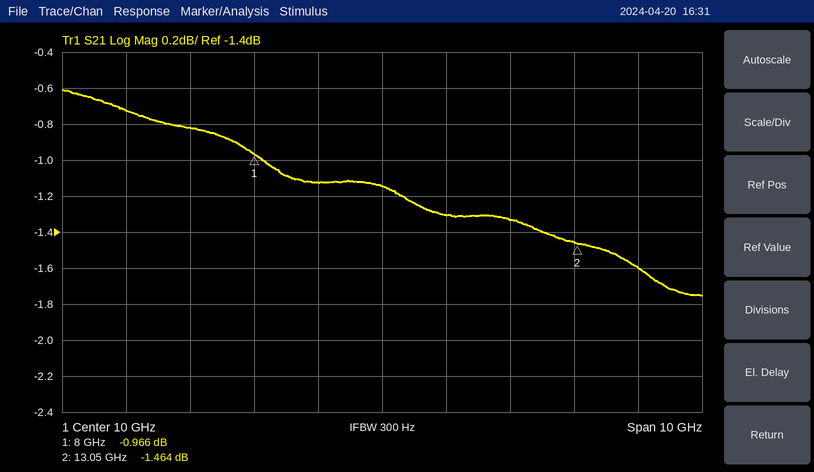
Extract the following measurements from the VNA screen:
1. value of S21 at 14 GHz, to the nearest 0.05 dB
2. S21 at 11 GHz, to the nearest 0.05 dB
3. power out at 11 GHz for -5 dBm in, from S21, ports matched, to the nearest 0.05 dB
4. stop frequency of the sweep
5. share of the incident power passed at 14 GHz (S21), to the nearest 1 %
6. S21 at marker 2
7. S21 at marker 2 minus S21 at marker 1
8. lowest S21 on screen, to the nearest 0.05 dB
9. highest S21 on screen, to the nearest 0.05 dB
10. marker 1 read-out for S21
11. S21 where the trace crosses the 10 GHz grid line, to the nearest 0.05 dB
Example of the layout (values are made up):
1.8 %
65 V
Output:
-1.60 dB
-1.30 dB
-6.30 dBm
15 GHz
69 %
-1.464 dB
-0.498 dB
-1.75 dB
-0.60 dB
-0.966 dB
-1.15 dB
